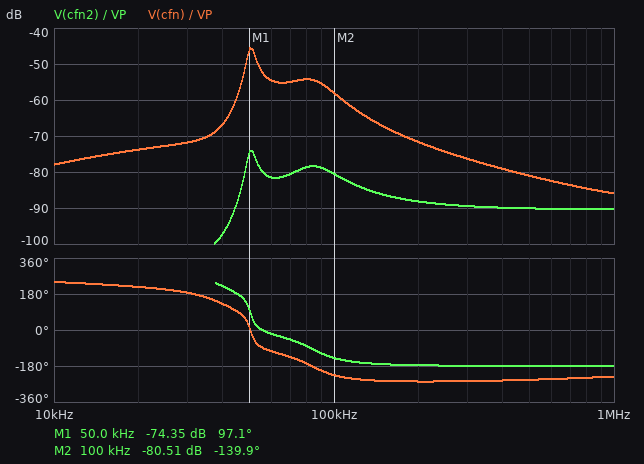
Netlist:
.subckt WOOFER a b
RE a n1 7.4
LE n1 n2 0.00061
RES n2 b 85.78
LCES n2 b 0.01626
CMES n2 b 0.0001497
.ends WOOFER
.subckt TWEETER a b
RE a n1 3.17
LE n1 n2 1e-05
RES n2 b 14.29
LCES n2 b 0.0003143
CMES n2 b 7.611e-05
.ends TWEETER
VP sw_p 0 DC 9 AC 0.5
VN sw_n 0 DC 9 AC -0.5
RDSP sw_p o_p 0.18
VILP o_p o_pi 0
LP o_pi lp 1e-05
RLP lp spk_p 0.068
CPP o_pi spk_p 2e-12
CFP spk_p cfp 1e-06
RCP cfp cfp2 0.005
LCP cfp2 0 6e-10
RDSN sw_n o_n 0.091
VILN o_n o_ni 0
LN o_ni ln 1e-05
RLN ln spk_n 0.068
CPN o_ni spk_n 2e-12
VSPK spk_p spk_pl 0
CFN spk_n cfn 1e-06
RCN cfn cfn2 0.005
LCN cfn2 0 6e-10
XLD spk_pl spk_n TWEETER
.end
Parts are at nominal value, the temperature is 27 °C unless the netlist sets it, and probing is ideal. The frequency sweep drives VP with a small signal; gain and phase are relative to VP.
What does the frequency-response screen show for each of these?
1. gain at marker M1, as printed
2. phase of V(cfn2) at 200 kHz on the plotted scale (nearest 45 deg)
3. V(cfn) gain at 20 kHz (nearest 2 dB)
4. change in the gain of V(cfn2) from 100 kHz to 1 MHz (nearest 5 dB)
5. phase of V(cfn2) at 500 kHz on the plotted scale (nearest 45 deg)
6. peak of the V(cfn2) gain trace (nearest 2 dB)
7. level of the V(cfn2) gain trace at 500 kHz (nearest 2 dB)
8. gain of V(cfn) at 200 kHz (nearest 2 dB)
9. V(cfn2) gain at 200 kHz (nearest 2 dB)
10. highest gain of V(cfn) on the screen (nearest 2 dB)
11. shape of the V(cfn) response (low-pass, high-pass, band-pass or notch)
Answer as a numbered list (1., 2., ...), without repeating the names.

1. -74.35 dB
2. -180 deg
3. -74 dB
4. -10 dB
5. -180 deg
6. -74 dB
7. -90 dB
8. -72 dB
9. -88 dB
10. -46 dB
11. band-pass
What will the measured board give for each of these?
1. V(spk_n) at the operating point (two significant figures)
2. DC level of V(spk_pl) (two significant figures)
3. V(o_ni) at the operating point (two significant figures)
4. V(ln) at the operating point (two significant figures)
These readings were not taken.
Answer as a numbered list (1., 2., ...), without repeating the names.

1. 9.0 V
2. 9.0 V
3. 9.0 V
4. 9.0 V
